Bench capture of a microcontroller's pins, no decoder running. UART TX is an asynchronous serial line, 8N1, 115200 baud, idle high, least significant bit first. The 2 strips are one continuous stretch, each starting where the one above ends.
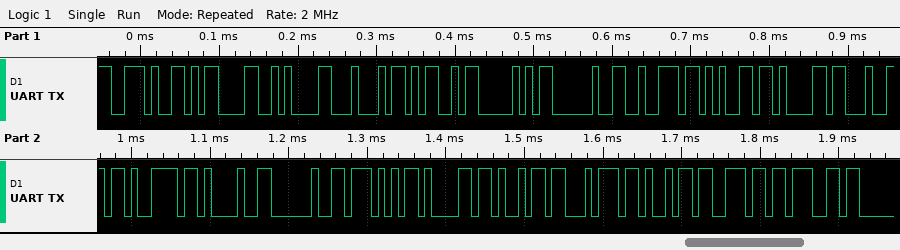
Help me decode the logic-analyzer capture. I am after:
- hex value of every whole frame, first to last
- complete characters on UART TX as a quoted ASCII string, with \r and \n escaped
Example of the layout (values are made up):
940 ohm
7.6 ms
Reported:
0x2E 0x0D 0x0A 0x44 0x4D 0x50 0x20 0x72 0x65 0x61 0x64 0x79 0x21 0x20 0x57 0x61 0x69 0x74 0x69 0x6E 0x67
".\r\nDMP ready! Waiting"
